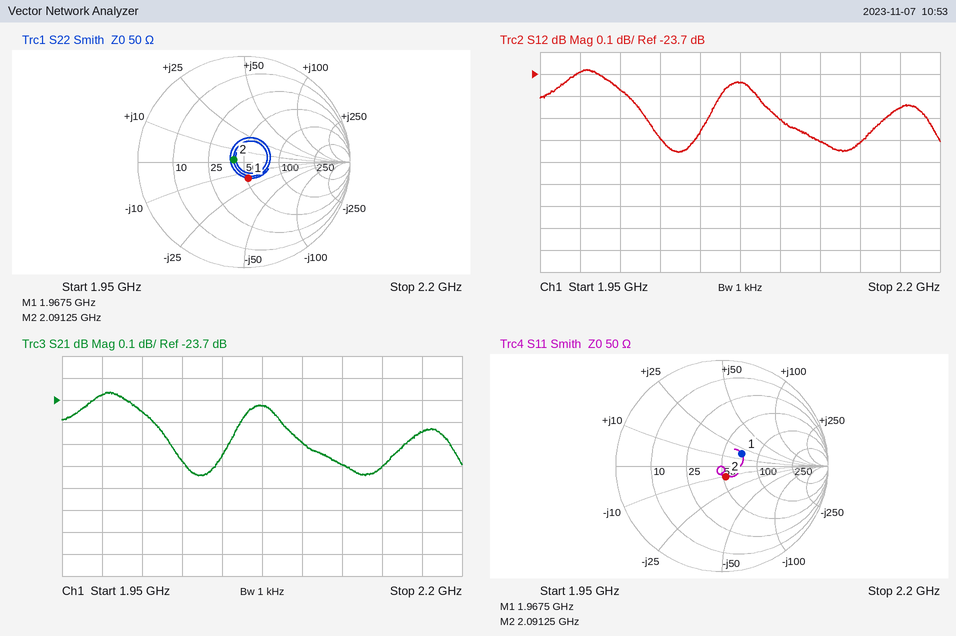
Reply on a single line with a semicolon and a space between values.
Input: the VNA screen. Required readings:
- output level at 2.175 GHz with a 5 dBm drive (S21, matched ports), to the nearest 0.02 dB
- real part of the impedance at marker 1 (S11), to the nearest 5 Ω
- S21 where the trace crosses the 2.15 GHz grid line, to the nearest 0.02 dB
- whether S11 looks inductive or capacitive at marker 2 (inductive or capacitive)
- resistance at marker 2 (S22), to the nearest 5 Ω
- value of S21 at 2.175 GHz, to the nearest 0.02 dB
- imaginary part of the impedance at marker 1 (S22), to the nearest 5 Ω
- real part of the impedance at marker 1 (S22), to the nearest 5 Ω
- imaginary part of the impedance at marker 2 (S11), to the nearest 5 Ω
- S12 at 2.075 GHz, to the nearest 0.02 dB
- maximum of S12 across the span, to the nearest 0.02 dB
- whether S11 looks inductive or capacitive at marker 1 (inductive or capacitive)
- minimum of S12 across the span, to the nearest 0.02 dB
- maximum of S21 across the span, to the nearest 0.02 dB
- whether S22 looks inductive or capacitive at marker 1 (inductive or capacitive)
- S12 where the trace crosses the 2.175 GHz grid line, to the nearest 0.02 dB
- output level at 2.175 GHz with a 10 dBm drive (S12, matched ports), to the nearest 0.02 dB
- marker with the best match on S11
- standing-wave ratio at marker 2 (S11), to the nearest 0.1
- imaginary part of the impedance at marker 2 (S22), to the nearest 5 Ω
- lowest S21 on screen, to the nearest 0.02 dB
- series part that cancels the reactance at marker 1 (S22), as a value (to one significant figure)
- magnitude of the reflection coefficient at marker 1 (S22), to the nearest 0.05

-18.84 dBm; 70 Ω; -24.00 dB; capacitive; 40 Ω; -23.84 dB; -15 Ω; 50 Ω; -10 Ω; -23.74 dB; -23.68 dB; inductive; -24.06 dB; -23.66 dB; capacitive; -23.86 dB; -13.86 dBm; marker 2; 1.2; 0 Ω; -24.04 dB; 1 nH; 0.15
